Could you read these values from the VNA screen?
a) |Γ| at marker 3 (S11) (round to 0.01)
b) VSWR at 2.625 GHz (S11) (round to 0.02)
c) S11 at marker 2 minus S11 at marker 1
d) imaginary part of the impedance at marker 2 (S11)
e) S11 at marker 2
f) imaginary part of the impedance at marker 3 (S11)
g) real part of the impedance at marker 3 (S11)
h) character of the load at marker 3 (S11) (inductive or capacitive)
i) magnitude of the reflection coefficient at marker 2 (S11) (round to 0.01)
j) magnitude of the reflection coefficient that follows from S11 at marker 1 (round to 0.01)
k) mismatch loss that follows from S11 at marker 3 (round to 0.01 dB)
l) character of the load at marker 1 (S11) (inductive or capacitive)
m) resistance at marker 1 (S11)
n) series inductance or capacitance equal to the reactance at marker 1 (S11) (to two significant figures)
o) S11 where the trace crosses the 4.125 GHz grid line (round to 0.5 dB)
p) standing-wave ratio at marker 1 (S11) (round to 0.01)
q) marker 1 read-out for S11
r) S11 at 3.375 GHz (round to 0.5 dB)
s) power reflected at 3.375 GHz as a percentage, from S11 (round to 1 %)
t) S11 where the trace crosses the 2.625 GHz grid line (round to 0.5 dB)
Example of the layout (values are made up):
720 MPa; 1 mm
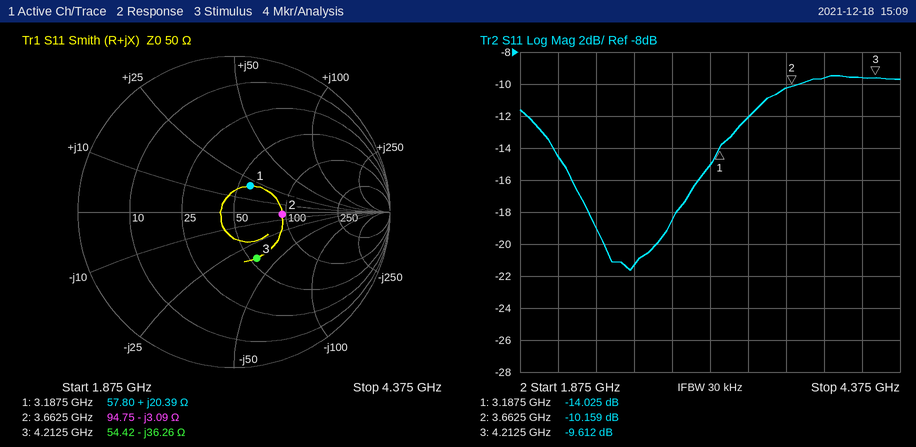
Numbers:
0.33; 1.18; 3.866 dB; -3.09 Ω; -10.159 dB; -36.26 Ω; 54.42 Ω; capacitive; 0.31; 0.20; 0.50 dB; inductive; 57.80 Ω; 1.0 nH; -9.5 dB; 1.50; -14.025 dB; -12.0 dB; 6 %; -21.5 dB
